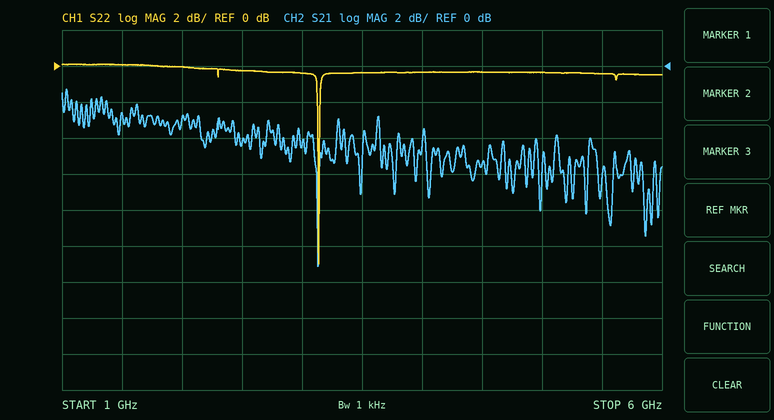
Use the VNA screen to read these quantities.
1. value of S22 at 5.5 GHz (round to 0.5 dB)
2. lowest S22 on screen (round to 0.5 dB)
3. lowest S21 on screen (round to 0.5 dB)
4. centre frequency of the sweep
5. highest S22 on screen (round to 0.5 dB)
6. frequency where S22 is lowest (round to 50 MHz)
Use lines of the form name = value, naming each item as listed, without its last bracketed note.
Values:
value of S22 at 5.5 GHz = -0.5 dB
lowest S22 on screen = -11.0 dB
lowest S21 on screen = -11.0 dB
centre frequency of the sweep = 3.5 GHz
highest S22 on screen = 0.0 dB
frequency where S22 is lowest = 3.15 GHz
